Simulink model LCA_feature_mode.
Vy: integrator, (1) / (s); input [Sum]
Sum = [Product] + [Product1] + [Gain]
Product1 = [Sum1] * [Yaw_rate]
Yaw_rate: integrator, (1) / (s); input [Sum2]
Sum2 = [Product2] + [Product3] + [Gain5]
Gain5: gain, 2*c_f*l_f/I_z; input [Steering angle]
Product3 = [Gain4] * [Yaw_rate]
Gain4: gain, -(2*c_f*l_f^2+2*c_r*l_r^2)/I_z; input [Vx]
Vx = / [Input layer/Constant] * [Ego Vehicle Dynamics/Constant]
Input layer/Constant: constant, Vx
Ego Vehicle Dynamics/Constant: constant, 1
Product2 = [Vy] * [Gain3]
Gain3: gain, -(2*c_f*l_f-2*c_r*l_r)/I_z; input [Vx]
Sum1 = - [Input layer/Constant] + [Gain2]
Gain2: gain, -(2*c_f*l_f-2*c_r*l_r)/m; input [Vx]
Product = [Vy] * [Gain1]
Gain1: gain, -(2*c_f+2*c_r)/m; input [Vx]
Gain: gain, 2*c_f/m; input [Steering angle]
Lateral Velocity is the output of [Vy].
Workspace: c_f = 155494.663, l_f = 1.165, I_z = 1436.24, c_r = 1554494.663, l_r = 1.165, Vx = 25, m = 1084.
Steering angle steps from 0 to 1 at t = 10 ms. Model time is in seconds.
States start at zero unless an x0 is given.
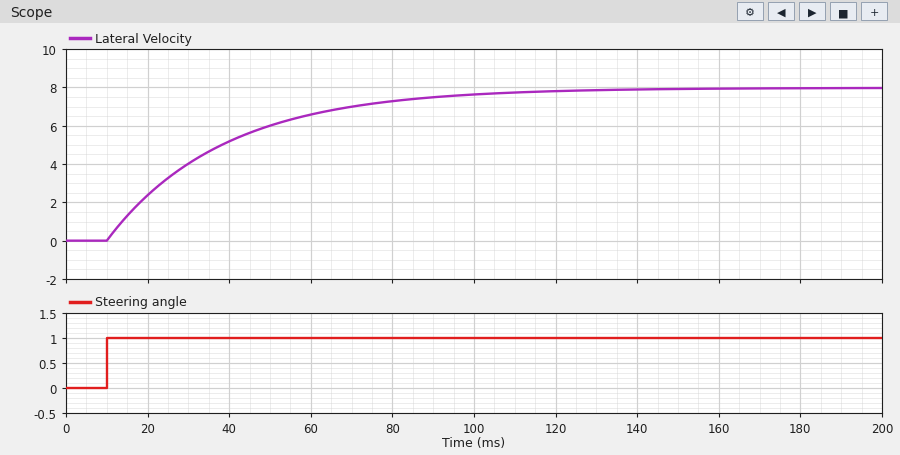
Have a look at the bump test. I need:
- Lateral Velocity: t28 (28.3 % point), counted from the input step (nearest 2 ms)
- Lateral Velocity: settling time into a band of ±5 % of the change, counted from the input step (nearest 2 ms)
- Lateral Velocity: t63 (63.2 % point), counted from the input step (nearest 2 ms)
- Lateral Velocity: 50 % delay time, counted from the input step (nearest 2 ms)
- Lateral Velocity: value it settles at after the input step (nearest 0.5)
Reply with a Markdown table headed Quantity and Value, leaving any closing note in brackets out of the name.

| Quantity | Value |
|---|---|
| Lateral Velocity: t28 (28.3 % point), counted from the input step | 10 ms |
| Lateral Velocity: settling time into a band of ±5 % of the change, counted from the input step | 86 ms |
| Lateral Velocity: t63 (63.2 % point), counted from the input step | 28 ms |
| Lateral Velocity: 50 % delay time, counted from the input step | 20 ms |
| Lateral Velocity: value it settles at after the input step | 8.0 |
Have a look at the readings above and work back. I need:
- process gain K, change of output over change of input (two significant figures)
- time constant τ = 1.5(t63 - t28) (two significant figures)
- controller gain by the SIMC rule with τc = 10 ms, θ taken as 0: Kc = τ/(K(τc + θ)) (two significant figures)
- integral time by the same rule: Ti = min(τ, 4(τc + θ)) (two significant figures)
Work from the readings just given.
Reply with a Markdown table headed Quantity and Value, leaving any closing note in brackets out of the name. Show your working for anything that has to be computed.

| Quantity | Value |
|---|---|
| process gain K, change of output over change of input | (8 - 0) / 1 = 8.0 |
| time constant τ = 1.5(t63 - t28) | 1.5 × (28 - 10) = 27 ms |
| controller gain by the SIMC rule with τc = 10 ms, θ taken as 0: Kc = τ/(K(τc + θ)) | 27 / (8 × (10 + 0)) = 0.34 |
| integral time by the same rule: Ti = min(τ, 4(τc + θ)) | min(27, 4 × (10 + 0)) = 27 ms |
